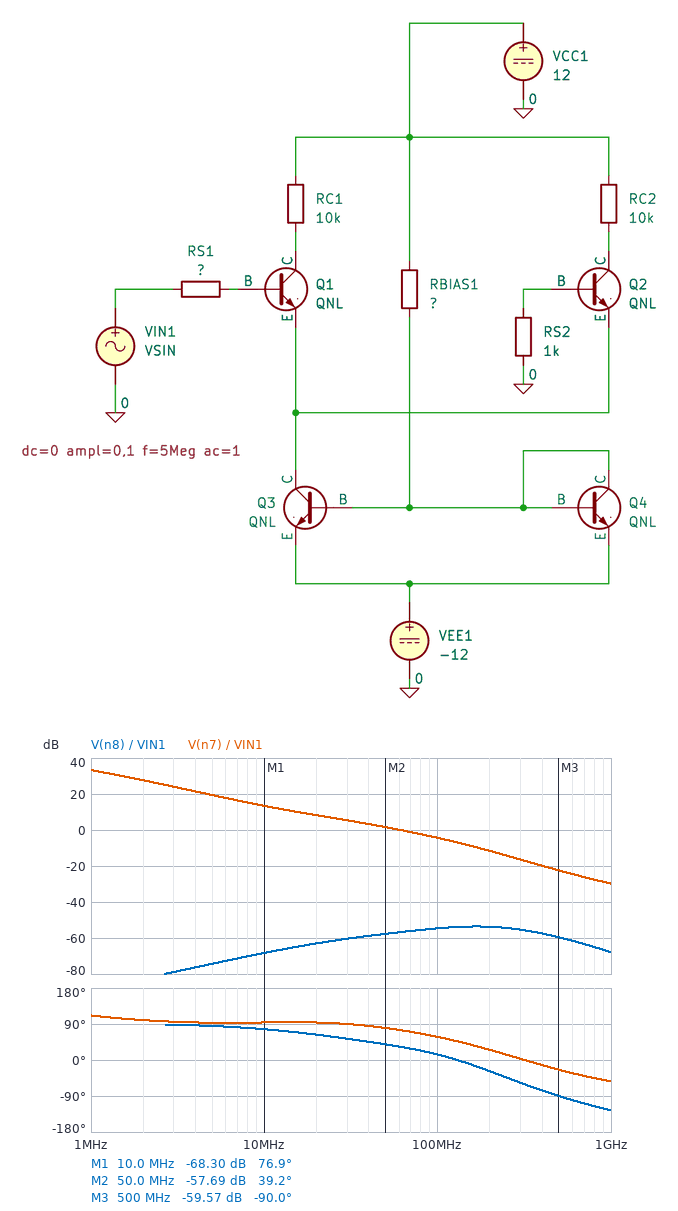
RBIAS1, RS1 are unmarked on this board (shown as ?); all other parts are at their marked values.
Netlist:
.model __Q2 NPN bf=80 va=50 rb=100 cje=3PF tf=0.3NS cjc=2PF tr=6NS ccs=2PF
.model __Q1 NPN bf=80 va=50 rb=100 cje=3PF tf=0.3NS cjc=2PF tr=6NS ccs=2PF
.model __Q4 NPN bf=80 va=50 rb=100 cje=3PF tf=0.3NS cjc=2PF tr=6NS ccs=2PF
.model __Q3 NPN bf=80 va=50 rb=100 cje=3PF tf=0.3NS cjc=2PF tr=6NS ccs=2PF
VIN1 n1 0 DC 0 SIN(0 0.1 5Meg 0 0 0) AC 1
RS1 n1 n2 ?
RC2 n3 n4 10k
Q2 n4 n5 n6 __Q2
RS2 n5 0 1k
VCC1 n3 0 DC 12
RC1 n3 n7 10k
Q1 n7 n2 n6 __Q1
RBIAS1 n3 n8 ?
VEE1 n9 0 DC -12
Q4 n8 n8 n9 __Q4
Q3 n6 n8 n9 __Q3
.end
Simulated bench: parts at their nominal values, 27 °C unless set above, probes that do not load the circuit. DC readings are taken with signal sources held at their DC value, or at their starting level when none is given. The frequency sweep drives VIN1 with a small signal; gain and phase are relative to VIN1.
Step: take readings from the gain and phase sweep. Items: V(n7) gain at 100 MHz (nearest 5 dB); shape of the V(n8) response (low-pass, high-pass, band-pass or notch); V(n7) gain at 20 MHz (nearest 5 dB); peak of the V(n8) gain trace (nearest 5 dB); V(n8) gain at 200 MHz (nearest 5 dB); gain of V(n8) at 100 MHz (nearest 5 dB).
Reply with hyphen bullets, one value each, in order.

- -5 dB
- band-pass
- 10 dB
- -55 dB
- -55 dB
- -55 dB
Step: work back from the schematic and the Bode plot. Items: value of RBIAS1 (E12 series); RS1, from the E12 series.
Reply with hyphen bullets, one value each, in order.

- 12 kΩ
- 560 Ω
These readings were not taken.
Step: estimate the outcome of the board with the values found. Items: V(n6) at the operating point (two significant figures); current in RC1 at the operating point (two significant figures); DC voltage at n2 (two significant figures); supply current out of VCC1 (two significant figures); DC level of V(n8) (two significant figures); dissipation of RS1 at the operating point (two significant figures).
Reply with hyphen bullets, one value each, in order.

- -790 mV
- 1.2 mA
- -8.4 mV
- 4.2 mA
- -11 V
- 130 nW
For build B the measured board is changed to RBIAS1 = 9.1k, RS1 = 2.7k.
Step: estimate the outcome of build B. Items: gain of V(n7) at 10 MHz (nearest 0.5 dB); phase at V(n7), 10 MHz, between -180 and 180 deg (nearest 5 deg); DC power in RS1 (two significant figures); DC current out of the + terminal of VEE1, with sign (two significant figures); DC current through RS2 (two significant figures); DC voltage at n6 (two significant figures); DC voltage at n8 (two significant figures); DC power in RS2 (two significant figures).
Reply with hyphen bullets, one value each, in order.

- -18.0 dB
- -35 deg
- 32 µW
- -5.5 mA
- 270 µA
- -1.1 V
- -11 V
- 75 µW
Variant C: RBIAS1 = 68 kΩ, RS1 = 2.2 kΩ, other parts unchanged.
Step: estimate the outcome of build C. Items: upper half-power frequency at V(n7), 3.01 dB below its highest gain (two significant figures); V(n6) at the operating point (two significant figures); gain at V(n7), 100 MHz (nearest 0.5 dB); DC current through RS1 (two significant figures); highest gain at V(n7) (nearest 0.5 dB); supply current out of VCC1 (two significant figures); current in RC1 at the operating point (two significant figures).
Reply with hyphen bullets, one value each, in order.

- 1.2 MHz
- -730 mV
- -12.0 dB
- 2.0 µA
- 30.5 dB
- 740 µA
- 190 µA
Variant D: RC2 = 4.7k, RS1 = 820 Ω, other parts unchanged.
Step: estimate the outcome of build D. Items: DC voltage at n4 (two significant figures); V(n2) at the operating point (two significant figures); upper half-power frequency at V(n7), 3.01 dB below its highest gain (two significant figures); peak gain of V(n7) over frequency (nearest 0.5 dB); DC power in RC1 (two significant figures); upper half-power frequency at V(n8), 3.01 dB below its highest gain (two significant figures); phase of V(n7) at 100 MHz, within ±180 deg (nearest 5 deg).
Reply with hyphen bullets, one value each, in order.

- 6.6 V
- -11 mV
- 590 kHz
- 42.0 dB
- 12 mW
- 340 MHz
- 55 deg
